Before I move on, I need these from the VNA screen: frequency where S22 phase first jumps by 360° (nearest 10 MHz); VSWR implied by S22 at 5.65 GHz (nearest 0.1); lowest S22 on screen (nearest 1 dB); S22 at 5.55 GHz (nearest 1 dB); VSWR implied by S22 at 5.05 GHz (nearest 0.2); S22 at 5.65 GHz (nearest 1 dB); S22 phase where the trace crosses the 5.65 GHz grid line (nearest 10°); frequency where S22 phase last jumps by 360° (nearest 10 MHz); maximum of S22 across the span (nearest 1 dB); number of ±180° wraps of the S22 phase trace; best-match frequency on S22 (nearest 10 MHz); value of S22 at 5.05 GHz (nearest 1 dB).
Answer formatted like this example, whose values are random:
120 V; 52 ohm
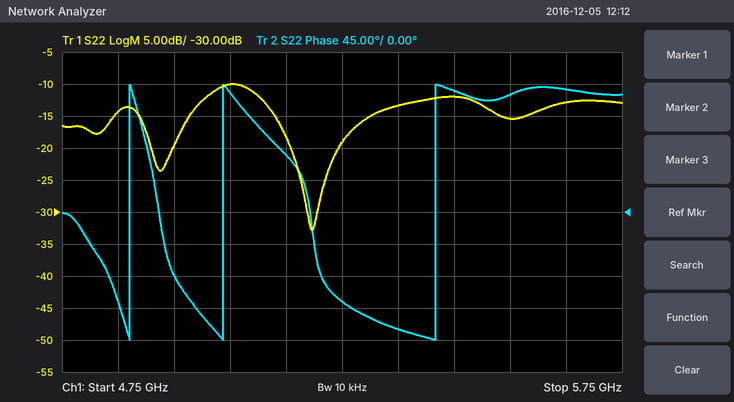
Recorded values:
4.87 GHz; 1.6; -33 dB; -15 dB; 2.0; -13 dB; 170°; 5.42 GHz; -10 dB; 3; 5.20 GHz; -10 dB
